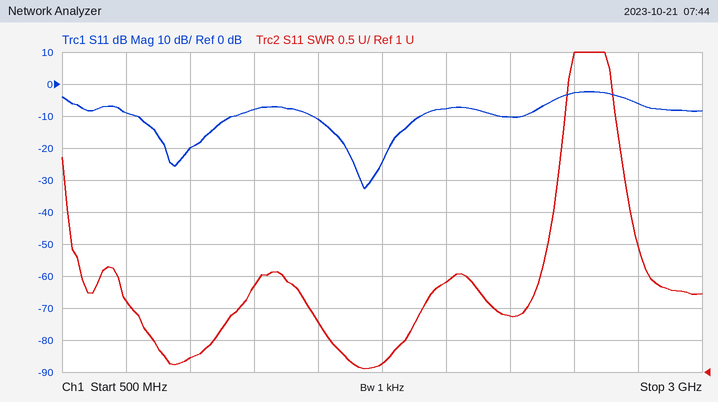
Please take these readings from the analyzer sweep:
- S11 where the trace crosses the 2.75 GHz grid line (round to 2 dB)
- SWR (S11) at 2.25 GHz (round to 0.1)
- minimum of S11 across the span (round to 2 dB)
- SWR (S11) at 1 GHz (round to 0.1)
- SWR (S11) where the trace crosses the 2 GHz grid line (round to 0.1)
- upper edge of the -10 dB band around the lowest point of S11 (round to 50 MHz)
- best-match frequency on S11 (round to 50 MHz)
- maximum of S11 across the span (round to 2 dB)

-6 dB
1.9
-32 dB
1.2
2.4
1.90 GHz
1.70 GHz
-2 dB
